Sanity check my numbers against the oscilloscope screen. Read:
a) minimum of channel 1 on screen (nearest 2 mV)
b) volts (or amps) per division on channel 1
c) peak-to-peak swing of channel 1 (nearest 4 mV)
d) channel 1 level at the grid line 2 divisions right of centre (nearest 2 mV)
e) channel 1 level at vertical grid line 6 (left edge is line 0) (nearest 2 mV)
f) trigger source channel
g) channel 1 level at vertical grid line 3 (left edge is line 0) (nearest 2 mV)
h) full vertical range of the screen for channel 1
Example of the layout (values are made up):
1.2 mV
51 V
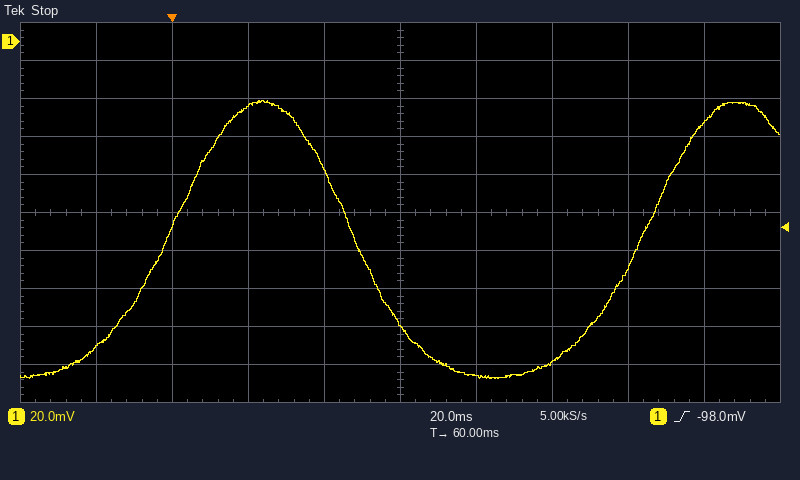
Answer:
-178 mV
20 mV
148 mV
-168 mV
-176 mV
channel 1
-34 mV
200 mV
